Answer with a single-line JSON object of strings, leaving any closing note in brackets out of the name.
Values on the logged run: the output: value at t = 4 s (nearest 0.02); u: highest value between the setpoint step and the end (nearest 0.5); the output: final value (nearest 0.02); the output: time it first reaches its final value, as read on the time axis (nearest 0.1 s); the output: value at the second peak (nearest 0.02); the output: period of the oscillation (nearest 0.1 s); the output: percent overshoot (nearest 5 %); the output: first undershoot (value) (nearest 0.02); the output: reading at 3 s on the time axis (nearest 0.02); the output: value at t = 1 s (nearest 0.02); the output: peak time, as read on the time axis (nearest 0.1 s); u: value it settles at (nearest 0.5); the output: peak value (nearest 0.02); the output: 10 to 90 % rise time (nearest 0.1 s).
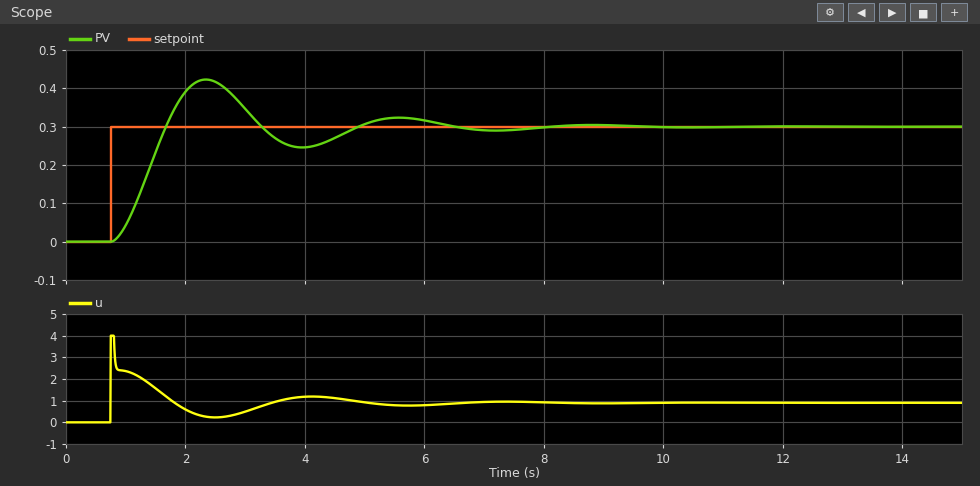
{"the output: value at t = 4 s": "0.24", "u: highest value between the setpoint step and the end": "4.0", "the output: final value": "0.30", "the output: time it first reaches its final value, as read on the time axis": "1.7 s", "the output: value at the second peak": "0.32", "the output: period of the oscillation": "3.2 s", "the output: percent overshoot": "40 %", "the output: first undershoot (value)": "0.24", "the output: reading at 3 s on the time axis": "0.34", "the output: value at t = 1 s": "0.04", "the output: peak time, as read on the time axis": "2.3 s", "u: value it settles at": "1.0", "the output: peak value": "0.42", "the output: 10 to 90 % rise time": "0.6 s"}
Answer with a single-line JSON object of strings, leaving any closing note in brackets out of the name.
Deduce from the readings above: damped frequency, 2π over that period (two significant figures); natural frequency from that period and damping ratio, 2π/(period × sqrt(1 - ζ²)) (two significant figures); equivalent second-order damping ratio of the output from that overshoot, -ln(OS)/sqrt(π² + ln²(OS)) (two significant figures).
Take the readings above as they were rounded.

{"damped frequency, 2π over that period": "2.0 rad/s", "natural frequency from that period and damping ratio, 2π/(period × sqrt(1 - ζ²))": "2.0 rad/s", "equivalent second-order damping ratio of the output from that overshoot, -ln(OS)/sqrt(π² + ln²(OS))": "0.28"}
